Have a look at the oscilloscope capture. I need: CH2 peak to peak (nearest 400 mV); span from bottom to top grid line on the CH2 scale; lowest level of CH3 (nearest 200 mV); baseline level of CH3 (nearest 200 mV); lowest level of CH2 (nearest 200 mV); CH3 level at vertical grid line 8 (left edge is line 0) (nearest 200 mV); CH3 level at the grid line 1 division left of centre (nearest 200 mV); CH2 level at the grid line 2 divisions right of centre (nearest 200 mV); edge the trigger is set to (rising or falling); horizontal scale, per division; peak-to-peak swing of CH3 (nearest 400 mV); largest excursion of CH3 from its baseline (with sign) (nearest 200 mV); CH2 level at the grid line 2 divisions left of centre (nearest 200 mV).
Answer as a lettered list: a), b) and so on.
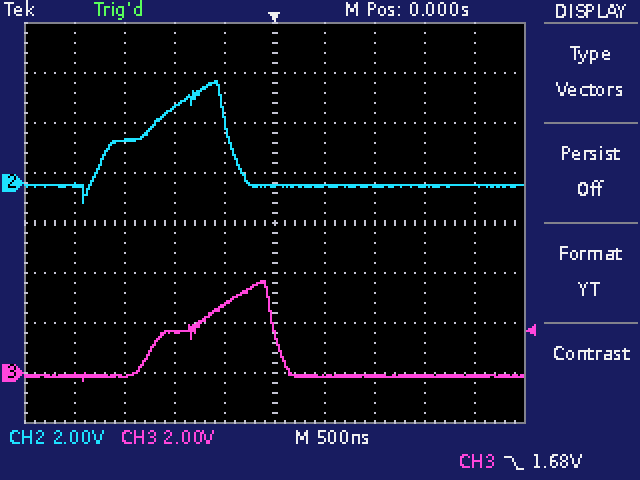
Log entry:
a) 4.8 V
b) 16 V
c) -400 mV
d) -200 mV
e) -800 mV
f) -200 mV
g) 2.8 V
h) -200 mV
i) falling
j) 500 ns
k) 4.0 V
l) +3.8 V
m) 3.0 V
